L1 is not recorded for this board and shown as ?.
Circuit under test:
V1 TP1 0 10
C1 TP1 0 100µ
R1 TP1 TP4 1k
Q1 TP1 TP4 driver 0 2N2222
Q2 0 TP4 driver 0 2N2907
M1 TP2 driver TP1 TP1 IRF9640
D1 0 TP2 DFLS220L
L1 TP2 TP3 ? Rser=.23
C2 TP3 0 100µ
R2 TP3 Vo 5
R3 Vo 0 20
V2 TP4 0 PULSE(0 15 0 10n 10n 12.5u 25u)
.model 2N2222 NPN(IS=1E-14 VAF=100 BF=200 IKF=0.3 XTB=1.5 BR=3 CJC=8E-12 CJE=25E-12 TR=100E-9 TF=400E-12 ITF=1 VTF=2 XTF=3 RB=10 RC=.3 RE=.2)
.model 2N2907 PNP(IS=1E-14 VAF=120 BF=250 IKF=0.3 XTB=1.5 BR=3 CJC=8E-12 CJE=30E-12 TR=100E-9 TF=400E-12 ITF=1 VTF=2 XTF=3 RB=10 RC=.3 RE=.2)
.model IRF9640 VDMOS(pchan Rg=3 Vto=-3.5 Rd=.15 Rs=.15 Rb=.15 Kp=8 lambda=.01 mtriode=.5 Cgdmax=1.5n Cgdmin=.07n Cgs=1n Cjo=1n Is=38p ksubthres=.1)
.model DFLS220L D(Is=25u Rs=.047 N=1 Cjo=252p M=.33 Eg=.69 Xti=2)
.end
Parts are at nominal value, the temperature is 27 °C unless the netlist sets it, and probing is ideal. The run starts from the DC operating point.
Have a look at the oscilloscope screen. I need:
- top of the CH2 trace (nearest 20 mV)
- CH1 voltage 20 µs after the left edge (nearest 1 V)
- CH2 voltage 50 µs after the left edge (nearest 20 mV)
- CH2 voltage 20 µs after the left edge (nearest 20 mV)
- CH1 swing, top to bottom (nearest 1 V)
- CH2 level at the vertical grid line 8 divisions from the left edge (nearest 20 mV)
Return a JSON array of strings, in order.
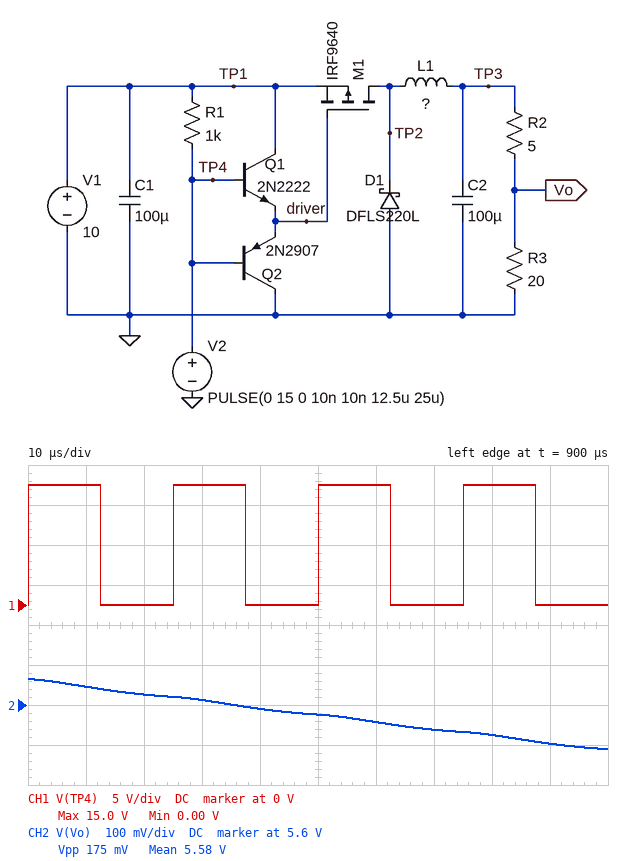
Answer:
["5.66 V", "0 V", "5.58 V", "5.62 V", "15 V", "5.52 V"]
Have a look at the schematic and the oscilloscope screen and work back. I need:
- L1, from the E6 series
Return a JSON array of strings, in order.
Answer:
["220 µH"]
